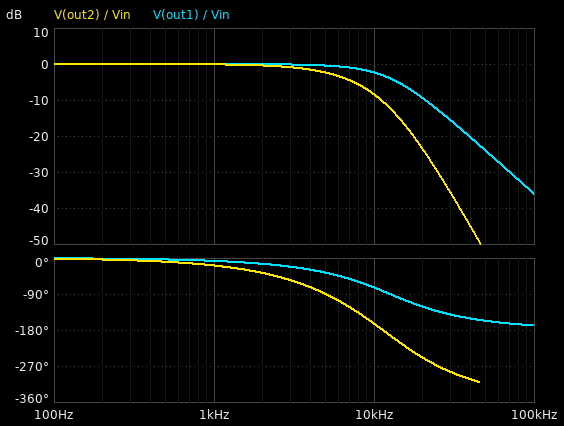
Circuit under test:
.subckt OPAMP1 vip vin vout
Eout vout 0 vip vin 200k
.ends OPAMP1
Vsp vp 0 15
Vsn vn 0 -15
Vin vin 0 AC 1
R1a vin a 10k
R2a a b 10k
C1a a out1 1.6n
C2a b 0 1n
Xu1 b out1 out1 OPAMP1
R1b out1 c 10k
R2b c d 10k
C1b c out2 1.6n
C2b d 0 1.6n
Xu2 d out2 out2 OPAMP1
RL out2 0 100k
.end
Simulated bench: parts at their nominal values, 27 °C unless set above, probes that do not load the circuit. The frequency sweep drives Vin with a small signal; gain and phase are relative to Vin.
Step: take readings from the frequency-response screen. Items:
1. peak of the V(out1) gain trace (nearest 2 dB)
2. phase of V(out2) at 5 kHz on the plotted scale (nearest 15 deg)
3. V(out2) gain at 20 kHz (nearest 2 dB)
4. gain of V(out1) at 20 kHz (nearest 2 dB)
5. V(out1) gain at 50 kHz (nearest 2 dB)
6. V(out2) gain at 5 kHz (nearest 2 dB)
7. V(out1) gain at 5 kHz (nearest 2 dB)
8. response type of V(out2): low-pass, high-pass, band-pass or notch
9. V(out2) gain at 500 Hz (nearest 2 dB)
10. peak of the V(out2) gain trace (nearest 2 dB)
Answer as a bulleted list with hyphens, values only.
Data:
- 0 dB
- -90 deg
- -24 dB
- -10 dB
- -24 dB
- -2 dB
- 0 dB
- low-pass
- 0 dB
- 0 dB
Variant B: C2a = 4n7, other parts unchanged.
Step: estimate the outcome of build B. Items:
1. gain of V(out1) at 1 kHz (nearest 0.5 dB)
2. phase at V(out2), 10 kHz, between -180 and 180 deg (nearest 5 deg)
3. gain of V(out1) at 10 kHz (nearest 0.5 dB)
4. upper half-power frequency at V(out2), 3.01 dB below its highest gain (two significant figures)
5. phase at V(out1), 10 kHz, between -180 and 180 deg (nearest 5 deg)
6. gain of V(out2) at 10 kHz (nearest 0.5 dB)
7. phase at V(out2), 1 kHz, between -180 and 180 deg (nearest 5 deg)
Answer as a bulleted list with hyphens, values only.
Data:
- -1.0 dB
- 160 deg
- -16.0 dB
- 1.7 kHz
- -110 deg
- -22.0 dB
- -45 deg
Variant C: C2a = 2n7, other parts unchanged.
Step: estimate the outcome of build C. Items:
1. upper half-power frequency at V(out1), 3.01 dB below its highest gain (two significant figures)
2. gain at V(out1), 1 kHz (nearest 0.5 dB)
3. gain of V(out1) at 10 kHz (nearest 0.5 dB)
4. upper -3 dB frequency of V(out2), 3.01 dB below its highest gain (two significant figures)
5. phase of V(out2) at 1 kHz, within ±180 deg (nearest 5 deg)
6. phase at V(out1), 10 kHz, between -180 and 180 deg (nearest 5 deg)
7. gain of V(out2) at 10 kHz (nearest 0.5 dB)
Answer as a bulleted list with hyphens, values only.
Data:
- 3.4 kHz
- -0.5 dB
- -11.0 dB
- 2.9 kHz
- -30 deg
- -100 deg
- -17.0 dB
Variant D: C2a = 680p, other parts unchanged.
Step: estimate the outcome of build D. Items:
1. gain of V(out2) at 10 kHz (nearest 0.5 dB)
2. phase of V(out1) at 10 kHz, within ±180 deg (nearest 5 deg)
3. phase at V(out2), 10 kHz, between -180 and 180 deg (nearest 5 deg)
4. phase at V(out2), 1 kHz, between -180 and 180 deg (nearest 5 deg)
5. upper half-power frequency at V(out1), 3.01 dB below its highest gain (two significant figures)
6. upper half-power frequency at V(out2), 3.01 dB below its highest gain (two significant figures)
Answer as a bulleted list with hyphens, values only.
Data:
- -6.5 dB
- -55 deg
- -145 deg
- -15 deg
- 16 kHz
- 6.5 kHz
